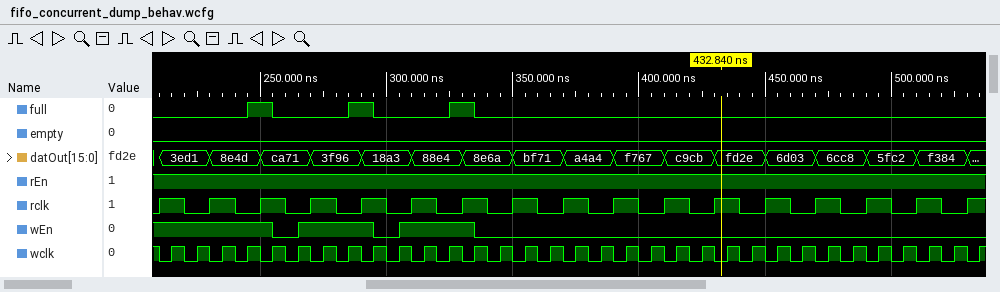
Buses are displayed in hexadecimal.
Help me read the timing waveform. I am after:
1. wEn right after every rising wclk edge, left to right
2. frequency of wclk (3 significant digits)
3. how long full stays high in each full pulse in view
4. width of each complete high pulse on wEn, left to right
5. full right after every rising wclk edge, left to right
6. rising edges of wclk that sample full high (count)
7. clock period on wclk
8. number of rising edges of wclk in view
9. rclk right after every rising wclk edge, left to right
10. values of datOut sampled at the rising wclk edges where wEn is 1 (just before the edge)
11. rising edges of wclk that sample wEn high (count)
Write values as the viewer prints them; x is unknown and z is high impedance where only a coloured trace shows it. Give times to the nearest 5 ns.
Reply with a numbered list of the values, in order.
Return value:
1. 1 1 1 1 0 1 1 1 0 1 1 1 0 0 0 0 0 0 0 0 0 0 0 0 0 0 0 0 0 0 0 0 0
2. 100 MHz
3. 10 ns, 10 ns, 10 ns
4. 30 ns, 30 ns
5. 0 0 0 1 0 0 0 1 0 0 0 1 0 0 0 0 0 0 0 0 0 0 0 0 0 0 0 0 0 0 0 0 0
6. 3
7. 10 ns
8. 33
9. 1 0 1 0 1 0 1 0 1 0 1 0 1 0 1 0 1 0 1 0 1 0 1 0 1 0 1 0 1 0 1 0 1
10. 3ed1, 3ed1, 8e4d, 8e4d, ca71, 3f96, 3f96, 18a3, 88e4, 88e4, 8e6a
11. 11
